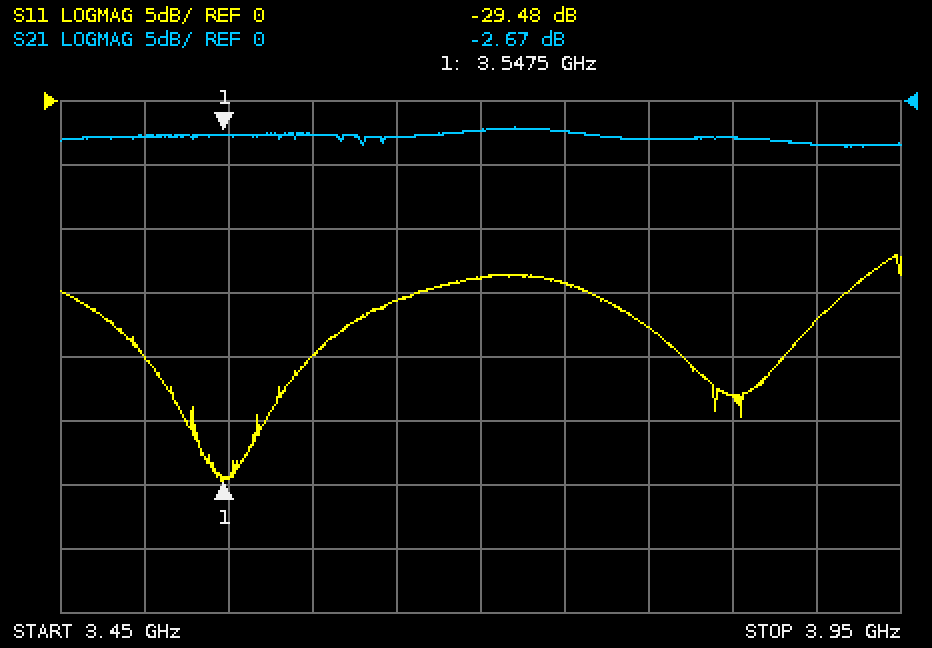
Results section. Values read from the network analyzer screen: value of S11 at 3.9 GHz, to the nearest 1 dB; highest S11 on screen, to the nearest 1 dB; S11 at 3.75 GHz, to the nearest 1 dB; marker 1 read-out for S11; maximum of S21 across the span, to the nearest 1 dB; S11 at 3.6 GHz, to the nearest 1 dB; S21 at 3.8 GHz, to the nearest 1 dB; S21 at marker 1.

-17 dB
-12 dB
-14 dB
-29.48 dB
-2 dB
-20 dB
-3 dB
-2.67 dB
